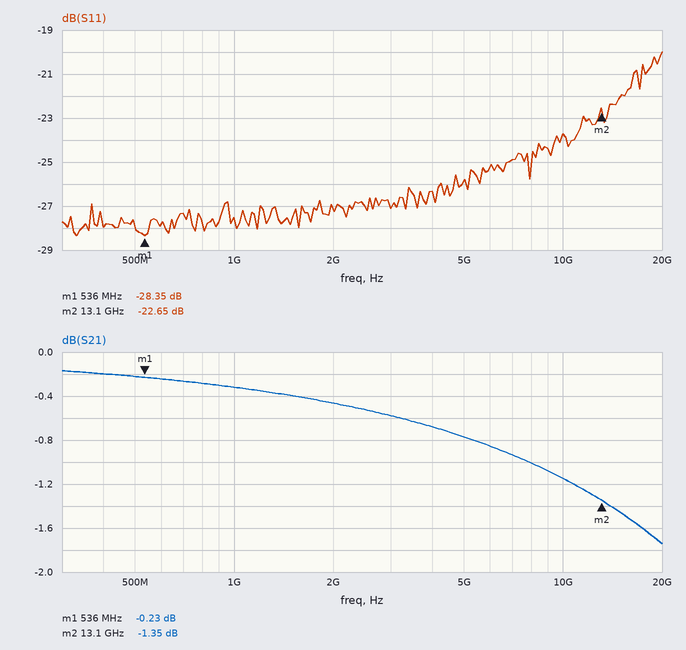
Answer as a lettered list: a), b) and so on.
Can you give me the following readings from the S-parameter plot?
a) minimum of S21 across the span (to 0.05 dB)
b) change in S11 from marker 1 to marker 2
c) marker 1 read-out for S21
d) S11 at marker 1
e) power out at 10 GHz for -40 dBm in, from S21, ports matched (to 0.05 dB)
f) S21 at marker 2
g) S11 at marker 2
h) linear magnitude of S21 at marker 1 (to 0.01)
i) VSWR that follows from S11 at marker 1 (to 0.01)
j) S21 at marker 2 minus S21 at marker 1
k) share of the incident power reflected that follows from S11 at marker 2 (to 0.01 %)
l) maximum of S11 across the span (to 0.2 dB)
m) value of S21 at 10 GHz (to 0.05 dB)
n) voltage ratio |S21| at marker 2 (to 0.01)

a) -1.75 dB
b) 5.70 dB
c) -0.23 dB
d) -28.35 dB
e) -41.15 dBm
f) -1.35 dB
g) -22.65 dB
h) 0.97
i) 1.08
j) -1.12 dB
k) 0.54 %
l) -20.0 dB
m) -1.15 dB
n) 0.86
